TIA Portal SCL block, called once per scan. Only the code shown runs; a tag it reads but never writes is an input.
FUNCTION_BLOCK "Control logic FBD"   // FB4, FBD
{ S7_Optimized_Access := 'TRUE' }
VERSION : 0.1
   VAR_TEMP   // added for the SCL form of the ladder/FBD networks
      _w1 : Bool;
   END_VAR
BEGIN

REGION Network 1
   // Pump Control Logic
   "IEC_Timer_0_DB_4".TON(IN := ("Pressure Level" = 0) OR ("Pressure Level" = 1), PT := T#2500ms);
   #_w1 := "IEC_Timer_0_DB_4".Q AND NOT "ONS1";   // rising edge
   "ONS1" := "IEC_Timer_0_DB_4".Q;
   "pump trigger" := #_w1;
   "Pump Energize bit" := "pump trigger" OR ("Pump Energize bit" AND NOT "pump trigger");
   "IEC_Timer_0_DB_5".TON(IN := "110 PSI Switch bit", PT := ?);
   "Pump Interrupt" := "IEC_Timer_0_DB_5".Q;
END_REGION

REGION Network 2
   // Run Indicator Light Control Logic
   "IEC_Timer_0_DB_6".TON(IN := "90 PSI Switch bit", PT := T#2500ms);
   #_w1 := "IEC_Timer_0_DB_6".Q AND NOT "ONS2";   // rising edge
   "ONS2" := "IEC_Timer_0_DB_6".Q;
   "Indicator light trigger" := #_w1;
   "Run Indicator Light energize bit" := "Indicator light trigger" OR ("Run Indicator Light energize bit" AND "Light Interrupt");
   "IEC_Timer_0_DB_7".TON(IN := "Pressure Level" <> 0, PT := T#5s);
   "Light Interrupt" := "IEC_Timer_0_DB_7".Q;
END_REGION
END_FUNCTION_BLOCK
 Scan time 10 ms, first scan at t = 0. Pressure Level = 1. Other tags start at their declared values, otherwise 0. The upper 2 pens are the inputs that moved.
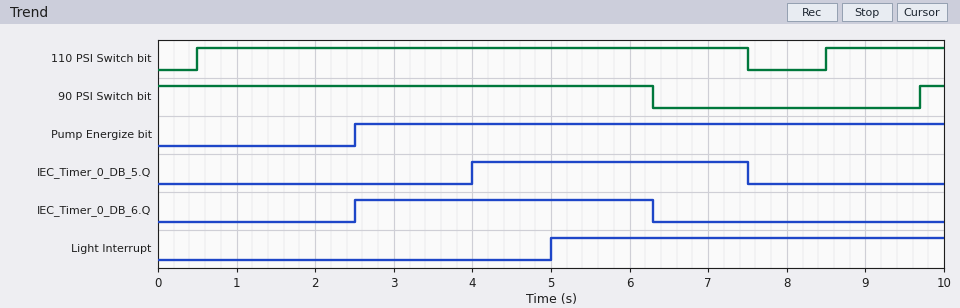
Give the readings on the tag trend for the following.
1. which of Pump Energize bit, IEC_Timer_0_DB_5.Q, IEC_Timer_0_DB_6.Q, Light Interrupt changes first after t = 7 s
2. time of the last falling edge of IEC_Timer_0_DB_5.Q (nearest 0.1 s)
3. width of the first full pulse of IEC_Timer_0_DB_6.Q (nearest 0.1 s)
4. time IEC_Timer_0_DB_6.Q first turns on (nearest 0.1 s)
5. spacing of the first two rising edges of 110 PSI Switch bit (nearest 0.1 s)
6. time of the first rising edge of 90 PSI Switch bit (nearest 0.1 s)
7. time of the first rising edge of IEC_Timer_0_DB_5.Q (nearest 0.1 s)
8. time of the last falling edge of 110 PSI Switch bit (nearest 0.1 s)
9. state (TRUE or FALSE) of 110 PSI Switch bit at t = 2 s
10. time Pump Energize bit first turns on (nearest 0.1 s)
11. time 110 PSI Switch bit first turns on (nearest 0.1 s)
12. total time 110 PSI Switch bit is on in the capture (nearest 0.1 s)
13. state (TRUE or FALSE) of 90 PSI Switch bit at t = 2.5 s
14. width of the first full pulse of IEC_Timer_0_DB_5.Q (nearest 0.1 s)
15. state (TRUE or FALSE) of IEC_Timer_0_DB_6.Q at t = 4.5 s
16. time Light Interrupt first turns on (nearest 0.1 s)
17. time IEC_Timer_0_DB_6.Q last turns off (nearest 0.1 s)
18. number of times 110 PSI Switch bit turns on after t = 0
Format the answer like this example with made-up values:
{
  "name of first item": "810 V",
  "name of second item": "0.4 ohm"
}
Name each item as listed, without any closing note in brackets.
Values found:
{
  "which of Pump Energize bit, IEC_Timer_0_DB_5.Q, IEC_Timer_0_DB_6.Q, Light Interrupt changes first after t = 7 s": "IEC_Timer_0_DB_5.Q",
  "time of the last falling edge of IEC_Timer_0_DB_5.Q": "7.5 s",
  "width of the first full pulse of IEC_Timer_0_DB_6.Q": "3.8 s",
  "time IEC_Timer_0_DB_6.Q first turns on": "2.5 s",
  "spacing of the first two rising edges of 110 PSI Switch bit": "8.0 s",
  "time of the first rising edge of 90 PSI Switch bit": "9.7 s",
  "time of the first rising edge of IEC_Timer_0_DB_5.Q": "4.0 s",
  "time of the last falling edge of 110 PSI Switch bit": "7.5 s",
  "state (TRUE or FALSE) of 110 PSI Switch bit at t = 2 s": "TRUE",
  "time Pump Energize bit first turns on": "2.5 s",
  "time 110 PSI Switch bit first turns on": "0.5 s",
  "total time 110 PSI Switch bit is on in the capture": "8.5 s",
  "state (TRUE or FALSE) of 90 PSI Switch bit at t = 2.5 s": "TRUE",
  "width of the first full pulse of IEC_Timer_0_DB_5.Q": "3.5 s",
  "state (TRUE or FALSE) of IEC_Timer_0_DB_6.Q at t = 4.5 s": "TRUE",
  "time Light Interrupt first turns on": "5.0 s",
  "time IEC_Timer_0_DB_6.Q last turns off": "6.3 s",
  "number of times 110 PSI Switch bit turns on after t = 0": "2"
}
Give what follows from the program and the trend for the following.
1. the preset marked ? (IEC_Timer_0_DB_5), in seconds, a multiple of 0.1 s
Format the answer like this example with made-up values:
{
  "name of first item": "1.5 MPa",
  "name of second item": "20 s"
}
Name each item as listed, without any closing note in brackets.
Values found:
{
  "the preset marked ? (IEC_Timer_0_DB_5), in seconds, a multiple of 0.1 s": "3.5 s"
}
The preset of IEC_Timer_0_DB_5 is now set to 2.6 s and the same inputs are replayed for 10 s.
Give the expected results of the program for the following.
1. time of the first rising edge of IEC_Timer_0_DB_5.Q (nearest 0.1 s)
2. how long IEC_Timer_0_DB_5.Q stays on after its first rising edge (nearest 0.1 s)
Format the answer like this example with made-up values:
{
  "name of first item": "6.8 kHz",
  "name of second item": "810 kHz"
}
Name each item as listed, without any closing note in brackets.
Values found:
{
  "time of the first rising edge of IEC_Timer_0_DB_5.Q": "3.1 s",
  "how long IEC_Timer_0_DB_5.Q stays on after its first rising edge": "4.4 s"
}
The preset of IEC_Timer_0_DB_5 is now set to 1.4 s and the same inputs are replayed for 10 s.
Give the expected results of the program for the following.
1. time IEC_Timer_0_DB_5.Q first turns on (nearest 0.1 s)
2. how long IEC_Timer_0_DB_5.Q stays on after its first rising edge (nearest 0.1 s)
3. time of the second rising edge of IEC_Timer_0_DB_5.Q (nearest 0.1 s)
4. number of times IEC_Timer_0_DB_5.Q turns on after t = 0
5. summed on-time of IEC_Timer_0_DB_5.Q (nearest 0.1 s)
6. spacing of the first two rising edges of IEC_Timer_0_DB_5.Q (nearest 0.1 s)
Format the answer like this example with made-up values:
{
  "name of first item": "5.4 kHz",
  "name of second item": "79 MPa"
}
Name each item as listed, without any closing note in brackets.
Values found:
{
  "time IEC_Timer_0_DB_5.Q first turns on": "1.9 s",
  "how long IEC_Timer_0_DB_5.Q stays on after its first rising edge": "5.6 s",
  "time of the second rising edge of IEC_Timer_0_DB_5.Q": "9.9 s",
  "number of times IEC_Timer_0_DB_5.Q turns on after t = 0": "2",
  "summed on-time of IEC_Timer_0_DB_5.Q": "5.7 s",
  "spacing of the first two rising edges of IEC_Timer_0_DB_5.Q": "8.0 s"
}
